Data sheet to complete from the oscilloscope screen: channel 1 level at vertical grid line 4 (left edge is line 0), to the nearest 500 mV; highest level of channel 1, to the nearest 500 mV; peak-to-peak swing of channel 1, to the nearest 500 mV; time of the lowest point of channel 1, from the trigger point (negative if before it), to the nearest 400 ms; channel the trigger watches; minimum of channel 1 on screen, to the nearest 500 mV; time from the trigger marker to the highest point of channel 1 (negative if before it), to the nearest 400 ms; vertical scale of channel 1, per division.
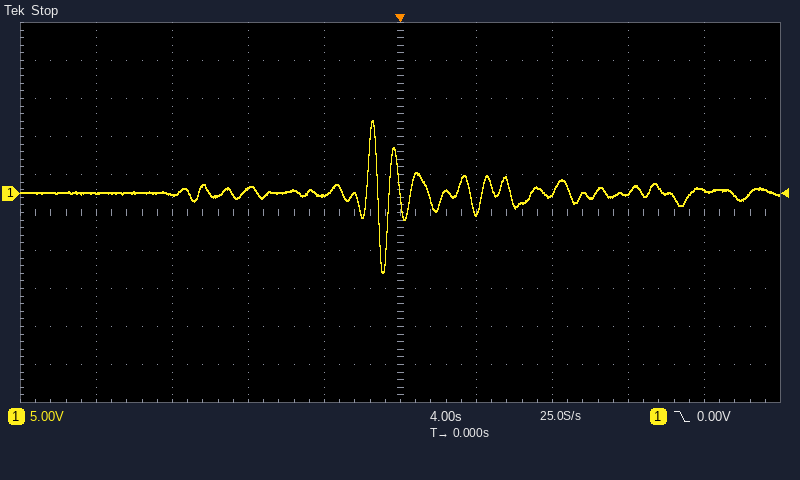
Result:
0.0 V
9.5 V
20.0 V
-800 ms
channel 1
-10.5 V
-1.6 s
5 V
